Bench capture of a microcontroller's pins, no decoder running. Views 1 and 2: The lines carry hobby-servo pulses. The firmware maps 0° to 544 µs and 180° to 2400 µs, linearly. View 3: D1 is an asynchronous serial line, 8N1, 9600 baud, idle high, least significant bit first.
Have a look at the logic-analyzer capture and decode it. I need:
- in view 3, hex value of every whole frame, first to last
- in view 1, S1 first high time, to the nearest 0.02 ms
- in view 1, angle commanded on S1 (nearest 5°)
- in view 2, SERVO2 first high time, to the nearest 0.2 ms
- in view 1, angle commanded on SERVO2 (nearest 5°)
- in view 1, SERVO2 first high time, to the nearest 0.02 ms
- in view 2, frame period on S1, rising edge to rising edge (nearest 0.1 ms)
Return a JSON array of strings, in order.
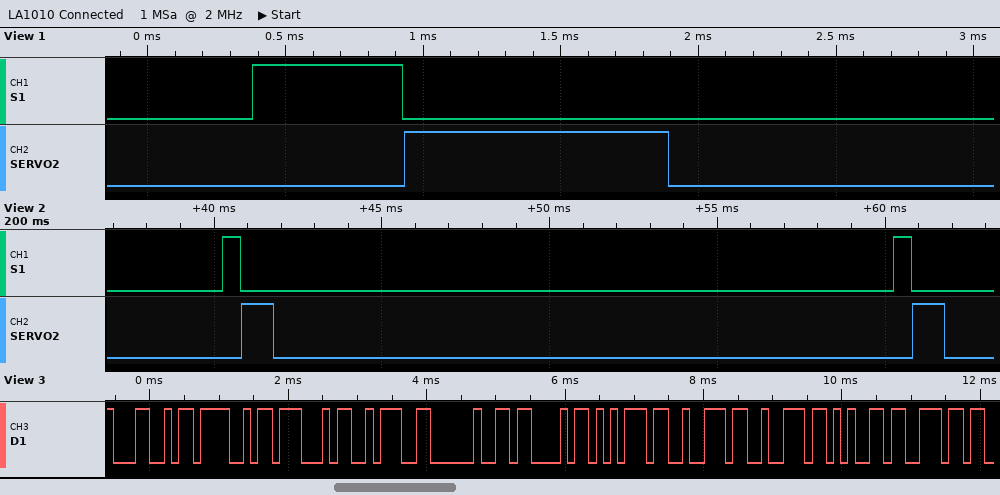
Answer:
["4C 4F 47 3A 20 43 75 72 72 65 6E", "0.54 ms", "0°", "1.0 ms", "40°", "0.96 ms", "20.0 ms"]
